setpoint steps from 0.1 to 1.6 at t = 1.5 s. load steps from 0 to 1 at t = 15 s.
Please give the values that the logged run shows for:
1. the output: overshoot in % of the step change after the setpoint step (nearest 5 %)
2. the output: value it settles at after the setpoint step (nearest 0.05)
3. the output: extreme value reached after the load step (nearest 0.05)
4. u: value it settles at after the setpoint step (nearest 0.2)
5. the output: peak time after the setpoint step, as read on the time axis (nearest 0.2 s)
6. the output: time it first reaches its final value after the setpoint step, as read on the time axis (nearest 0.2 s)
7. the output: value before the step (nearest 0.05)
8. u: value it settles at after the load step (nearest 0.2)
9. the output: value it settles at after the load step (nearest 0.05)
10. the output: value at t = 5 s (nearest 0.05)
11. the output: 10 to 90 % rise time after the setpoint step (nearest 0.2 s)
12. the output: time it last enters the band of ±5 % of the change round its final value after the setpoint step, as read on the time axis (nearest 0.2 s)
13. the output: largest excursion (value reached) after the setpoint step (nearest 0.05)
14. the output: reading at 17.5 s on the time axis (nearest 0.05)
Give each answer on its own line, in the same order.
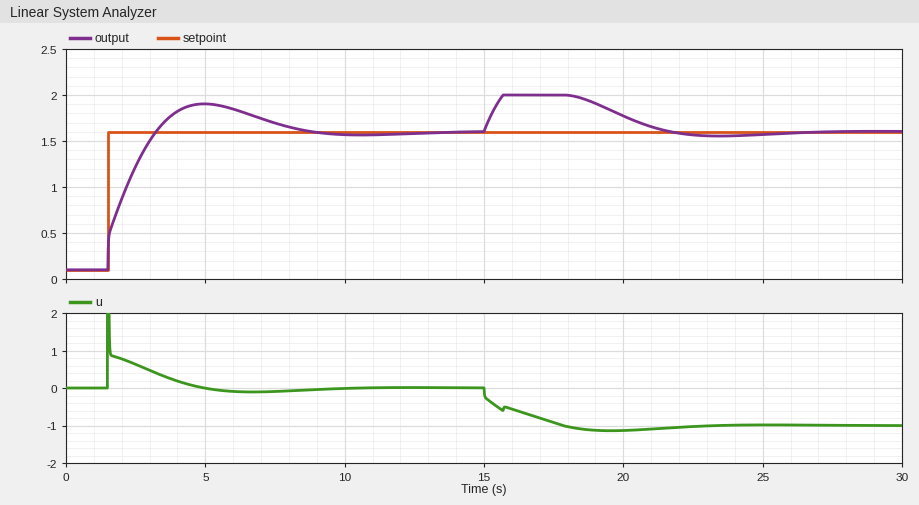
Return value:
20 %
1.60
2.00
0.0
5.0 s
3.2 s
0.10
-1.0
1.60
1.90
1.4 s
7.8 s
1.90
2.00
